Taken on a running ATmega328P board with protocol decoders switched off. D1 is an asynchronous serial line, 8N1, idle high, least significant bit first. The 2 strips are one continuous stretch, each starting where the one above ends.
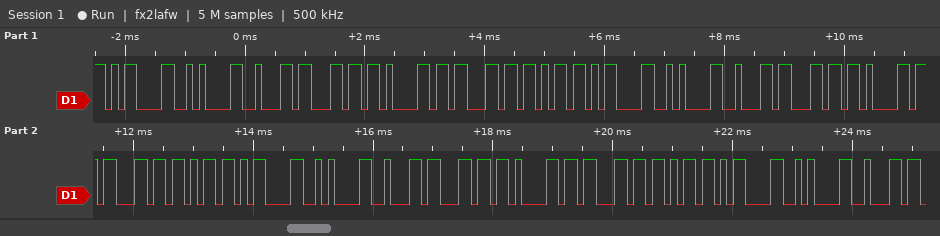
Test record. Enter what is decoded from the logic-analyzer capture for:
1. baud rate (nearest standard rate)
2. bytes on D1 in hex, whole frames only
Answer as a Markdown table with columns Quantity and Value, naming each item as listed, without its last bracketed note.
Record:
| Quantity | Value |
|---|---|
| baud rate | 9600 baud |
| bytes on D1 in hex, whole frames only | 0D 0A 62 6C 61 63 6B 0D 0A 62 6C 61 63 6B 0D 0A 62 6C 61 63 6B 0D 0A 62 |
